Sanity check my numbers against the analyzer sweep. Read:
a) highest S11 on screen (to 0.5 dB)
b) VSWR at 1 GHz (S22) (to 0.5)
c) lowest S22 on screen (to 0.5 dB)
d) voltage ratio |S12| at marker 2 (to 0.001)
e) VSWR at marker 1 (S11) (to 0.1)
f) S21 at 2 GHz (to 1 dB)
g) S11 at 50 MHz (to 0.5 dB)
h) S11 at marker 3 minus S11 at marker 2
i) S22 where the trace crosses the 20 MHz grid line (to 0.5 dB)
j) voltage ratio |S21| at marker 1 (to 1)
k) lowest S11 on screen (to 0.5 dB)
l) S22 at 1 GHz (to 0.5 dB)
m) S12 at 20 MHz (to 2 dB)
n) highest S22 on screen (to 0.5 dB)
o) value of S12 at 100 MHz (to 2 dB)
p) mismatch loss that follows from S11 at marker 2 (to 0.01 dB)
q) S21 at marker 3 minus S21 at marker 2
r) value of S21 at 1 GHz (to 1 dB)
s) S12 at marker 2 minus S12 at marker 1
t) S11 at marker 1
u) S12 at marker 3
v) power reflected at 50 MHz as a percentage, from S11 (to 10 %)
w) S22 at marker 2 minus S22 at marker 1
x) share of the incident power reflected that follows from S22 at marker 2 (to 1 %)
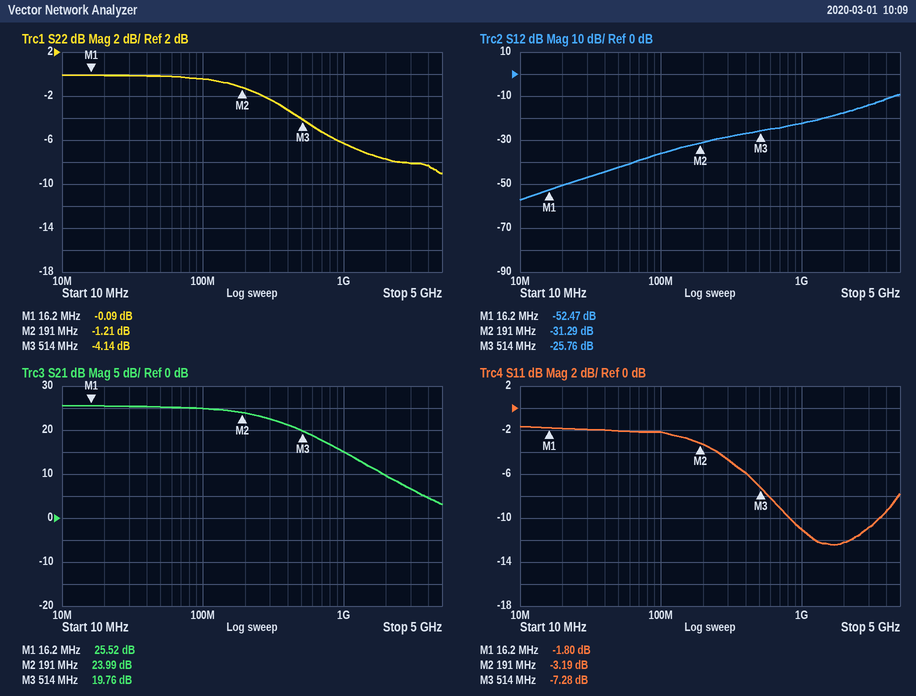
-1.5 dB
3.0
-9.0 dB
0.027
9.7
10 dB
-2.0 dB
-4.09 dB
0.0 dB
19
-12.5 dB
-6.5 dB
-50 dB
0.0 dB
-36 dB
2.84 dB
-4.23 dB
15 dB
21.18 dB
-1.80 dB
-25.76 dB
60 %
-1.12 dB
76 %
